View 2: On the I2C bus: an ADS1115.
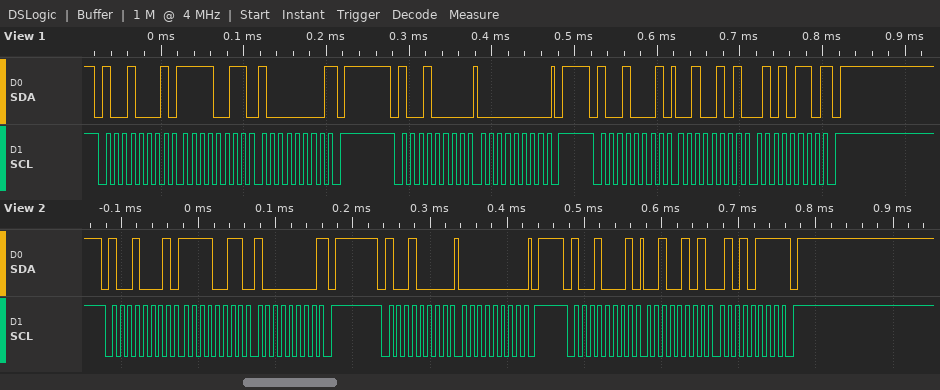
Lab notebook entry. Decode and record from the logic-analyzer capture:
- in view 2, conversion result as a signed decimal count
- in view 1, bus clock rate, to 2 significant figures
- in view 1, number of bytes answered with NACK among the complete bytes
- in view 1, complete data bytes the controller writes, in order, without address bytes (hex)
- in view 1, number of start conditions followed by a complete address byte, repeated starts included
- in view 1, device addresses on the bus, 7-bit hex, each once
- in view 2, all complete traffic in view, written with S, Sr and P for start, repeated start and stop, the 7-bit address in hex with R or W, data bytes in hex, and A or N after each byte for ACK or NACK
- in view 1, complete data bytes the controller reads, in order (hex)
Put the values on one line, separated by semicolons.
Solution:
9559; 100 kHz; 2; 00; 3; 0x48; S 48R A F3 A 80 N P S 48W A 00 A P S 48R A 25 A 57 N P; F3 80 25 56
